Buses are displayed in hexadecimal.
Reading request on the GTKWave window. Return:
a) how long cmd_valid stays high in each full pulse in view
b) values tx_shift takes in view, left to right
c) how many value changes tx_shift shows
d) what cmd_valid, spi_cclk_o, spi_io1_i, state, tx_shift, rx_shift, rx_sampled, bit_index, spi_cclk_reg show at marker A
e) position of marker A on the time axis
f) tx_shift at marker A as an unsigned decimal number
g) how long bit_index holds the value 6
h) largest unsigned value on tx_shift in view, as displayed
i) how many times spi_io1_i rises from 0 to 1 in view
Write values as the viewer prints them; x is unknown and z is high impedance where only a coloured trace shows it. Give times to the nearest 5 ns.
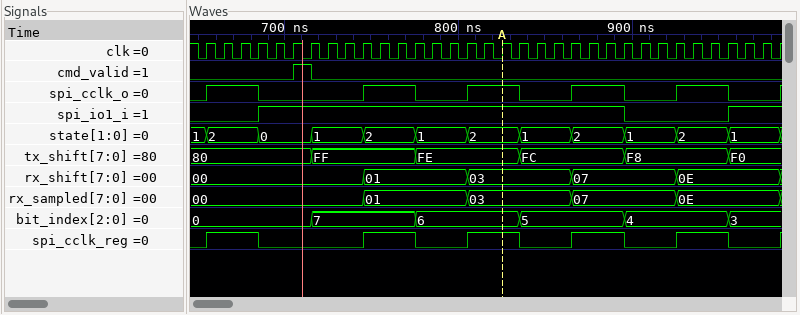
10 ns
80, FF, FE, FC, F8, F0
5
cmd_valid=0, spi_cclk_o=1, spi_io1_i=1, state=2, tx_shift=FE, rx_shift=03, rx_sampled=03, bit_index=6, spi_cclk_reg=1
825 ns
254
60 ns
FF
2
